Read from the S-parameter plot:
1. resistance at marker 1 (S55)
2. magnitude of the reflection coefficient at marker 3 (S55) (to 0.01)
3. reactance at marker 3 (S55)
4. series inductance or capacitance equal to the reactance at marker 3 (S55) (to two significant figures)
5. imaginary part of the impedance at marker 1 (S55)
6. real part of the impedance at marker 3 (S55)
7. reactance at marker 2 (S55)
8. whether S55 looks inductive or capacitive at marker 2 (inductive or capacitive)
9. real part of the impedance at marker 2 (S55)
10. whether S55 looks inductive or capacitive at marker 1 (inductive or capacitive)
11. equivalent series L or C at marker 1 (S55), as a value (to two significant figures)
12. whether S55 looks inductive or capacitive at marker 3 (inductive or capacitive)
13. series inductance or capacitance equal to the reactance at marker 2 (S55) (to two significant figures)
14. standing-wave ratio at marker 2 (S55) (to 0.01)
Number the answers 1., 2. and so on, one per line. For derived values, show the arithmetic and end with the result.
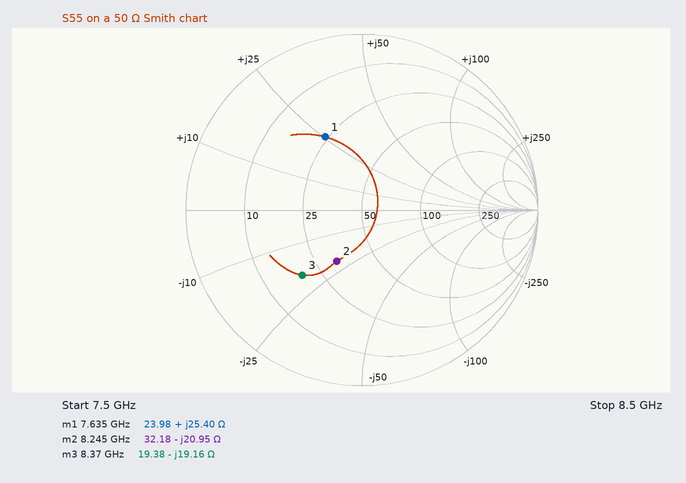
1. 23.98 Ω
2. 0.50
3. -19.16 Ω
4. C = 1/(2π × 8.37 GHz × 19.16 Ω) ≈ 992 fF, so 990 fF to two significant figures
5. +25.40 Ω
6. 19.38 Ω
7. -20.95 Ω
8. capacitive
9. 32.18 Ω
10. inductive
11. L = 25.4 Ω/(2π × 7.635 GHz) ≈ 529 pH, so 530 pH to two significant figures
12. capacitive
13. C = 1/(2π × 8.245 GHz × 20.95 Ω) ≈ 921 fF, so 920 fF to two significant figures
14. 1.96
